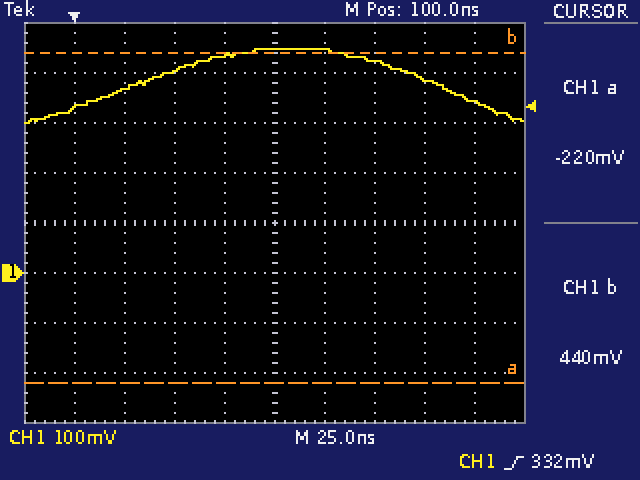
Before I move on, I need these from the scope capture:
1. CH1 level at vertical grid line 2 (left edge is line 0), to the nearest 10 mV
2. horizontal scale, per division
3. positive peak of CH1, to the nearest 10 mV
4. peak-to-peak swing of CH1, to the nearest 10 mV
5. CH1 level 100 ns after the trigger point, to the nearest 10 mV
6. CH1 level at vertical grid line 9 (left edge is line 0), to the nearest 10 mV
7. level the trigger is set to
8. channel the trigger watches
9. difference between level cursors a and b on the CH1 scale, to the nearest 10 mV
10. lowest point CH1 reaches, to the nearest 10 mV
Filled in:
370 mV
25 ns
450 mV
150 mV
450 mV
340 mV
332 mV
CH1
660 mV
300 mV
